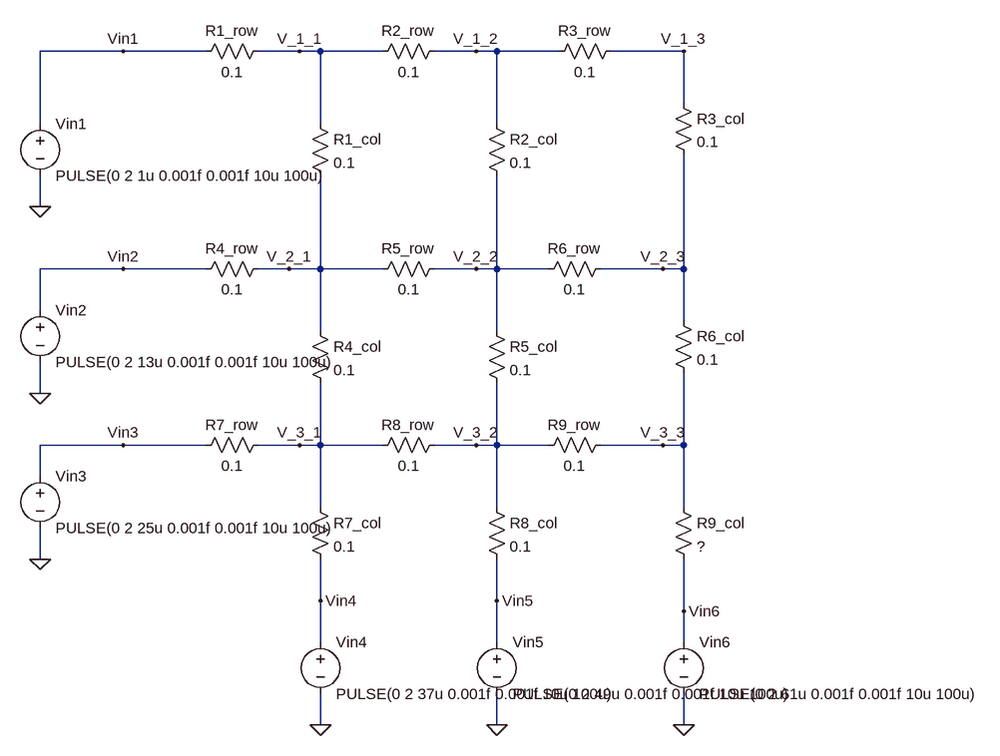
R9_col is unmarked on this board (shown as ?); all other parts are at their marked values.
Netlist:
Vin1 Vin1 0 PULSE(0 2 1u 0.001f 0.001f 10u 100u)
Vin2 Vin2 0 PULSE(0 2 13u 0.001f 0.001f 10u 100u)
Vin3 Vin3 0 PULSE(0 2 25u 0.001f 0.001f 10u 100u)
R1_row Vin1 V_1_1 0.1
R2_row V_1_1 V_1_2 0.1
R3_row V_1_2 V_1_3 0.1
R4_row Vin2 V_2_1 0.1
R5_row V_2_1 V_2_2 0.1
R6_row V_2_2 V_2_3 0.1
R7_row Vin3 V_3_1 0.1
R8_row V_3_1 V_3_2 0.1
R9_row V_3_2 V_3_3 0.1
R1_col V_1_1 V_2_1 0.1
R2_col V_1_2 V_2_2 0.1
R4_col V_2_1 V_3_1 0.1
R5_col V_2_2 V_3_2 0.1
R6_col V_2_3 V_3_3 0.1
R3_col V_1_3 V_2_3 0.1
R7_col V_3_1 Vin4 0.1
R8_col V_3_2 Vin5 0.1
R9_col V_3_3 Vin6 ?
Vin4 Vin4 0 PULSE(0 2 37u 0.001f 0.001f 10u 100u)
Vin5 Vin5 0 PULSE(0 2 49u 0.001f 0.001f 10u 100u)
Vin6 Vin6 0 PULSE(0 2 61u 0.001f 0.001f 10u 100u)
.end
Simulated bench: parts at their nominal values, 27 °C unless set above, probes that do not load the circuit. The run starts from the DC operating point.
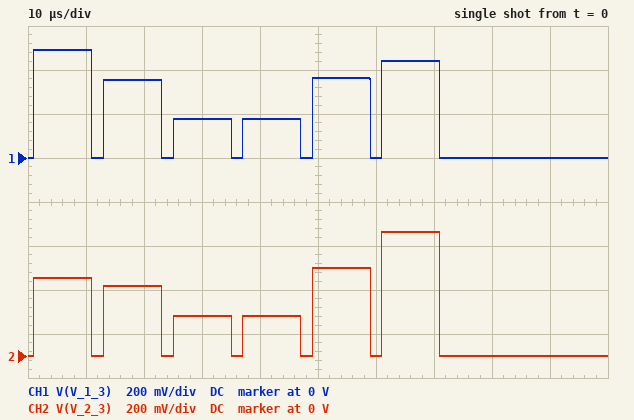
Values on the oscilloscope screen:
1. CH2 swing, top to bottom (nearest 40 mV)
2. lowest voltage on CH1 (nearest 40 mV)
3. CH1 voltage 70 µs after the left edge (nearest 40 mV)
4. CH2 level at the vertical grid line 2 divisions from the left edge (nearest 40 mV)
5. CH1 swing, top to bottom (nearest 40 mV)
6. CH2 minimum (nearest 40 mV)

560 mV
0 V
440 mV
320 mV
480 mV
0 V
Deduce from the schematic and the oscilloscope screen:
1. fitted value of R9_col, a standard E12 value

0.12 Ω
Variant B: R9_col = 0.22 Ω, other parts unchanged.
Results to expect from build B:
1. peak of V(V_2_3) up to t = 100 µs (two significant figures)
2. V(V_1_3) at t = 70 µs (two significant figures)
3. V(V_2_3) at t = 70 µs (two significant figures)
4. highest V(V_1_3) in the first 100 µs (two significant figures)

470 mV
300 mV
390 mV
510 mV
